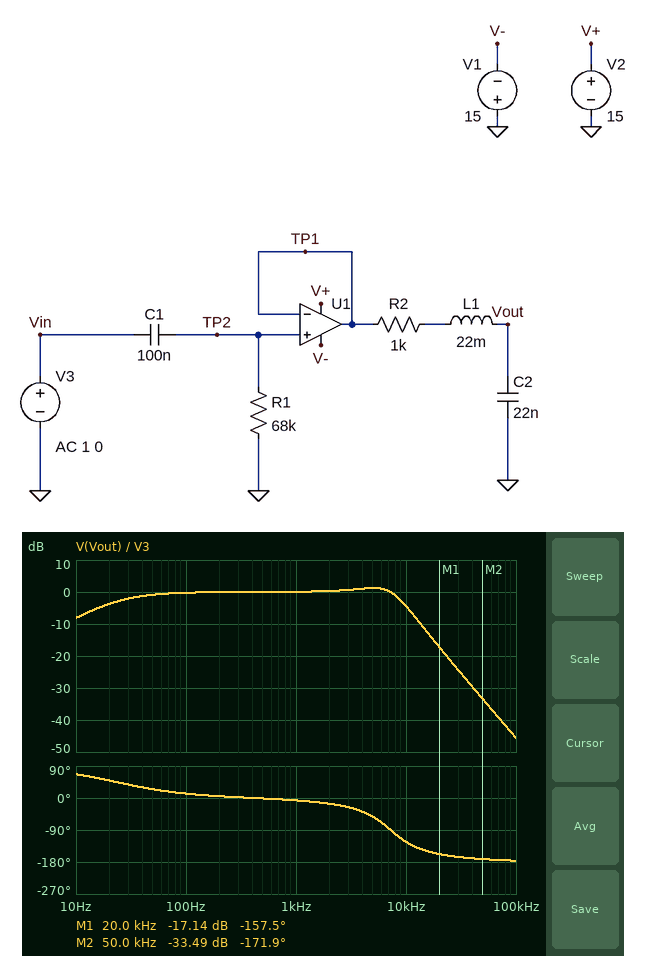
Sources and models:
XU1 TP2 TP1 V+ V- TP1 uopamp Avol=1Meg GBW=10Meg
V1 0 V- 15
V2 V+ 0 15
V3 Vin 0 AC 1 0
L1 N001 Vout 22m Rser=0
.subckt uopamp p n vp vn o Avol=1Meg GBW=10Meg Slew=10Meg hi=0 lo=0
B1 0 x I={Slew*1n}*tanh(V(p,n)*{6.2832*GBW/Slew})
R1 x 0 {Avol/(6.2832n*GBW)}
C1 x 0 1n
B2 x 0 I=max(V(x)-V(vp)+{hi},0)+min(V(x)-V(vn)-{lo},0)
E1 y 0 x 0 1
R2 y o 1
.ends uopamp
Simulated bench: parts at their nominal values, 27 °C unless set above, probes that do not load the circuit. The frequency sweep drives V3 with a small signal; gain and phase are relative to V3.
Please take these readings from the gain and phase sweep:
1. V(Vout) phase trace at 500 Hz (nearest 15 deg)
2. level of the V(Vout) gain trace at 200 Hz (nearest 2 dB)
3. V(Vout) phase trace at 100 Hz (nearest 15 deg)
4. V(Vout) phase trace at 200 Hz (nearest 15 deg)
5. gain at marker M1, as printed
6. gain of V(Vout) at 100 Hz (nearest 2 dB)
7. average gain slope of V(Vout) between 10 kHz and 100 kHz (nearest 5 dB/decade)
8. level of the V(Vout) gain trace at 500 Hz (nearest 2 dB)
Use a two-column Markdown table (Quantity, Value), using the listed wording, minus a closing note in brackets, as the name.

| Quantity | Value |
|---|---|
| V(Vout) phase trace at 500 Hz | 0 deg |
| level of the V(Vout) gain trace at 200 Hz | 0 dB |
| V(Vout) phase trace at 100 Hz | 15 deg |
| V(Vout) phase trace at 200 Hz | 0 deg |
| gain at marker M1, as printed | -17.14 dB |
| gain of V(Vout) at 100 Hz | 0 dB |
| average gain slope of V(Vout) between 10 kHz and 100 kHz | -40 dB/decade |
| level of the V(Vout) gain trace at 500 Hz | 0 dB |
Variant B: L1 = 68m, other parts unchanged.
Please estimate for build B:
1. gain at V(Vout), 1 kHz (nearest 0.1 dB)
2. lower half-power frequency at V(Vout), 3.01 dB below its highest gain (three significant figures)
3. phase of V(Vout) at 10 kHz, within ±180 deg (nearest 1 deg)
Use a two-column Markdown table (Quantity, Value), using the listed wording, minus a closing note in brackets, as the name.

| Quantity | Value |
|---|---|
| gain at V(Vout), 1 kHz | 0.4 dB |
| lower half-power frequency at V(Vout), 3.01 dB below its highest gain | 2.23 kHz |
| phase of V(Vout) at 10 kHz, within ±180 deg | -164 deg |
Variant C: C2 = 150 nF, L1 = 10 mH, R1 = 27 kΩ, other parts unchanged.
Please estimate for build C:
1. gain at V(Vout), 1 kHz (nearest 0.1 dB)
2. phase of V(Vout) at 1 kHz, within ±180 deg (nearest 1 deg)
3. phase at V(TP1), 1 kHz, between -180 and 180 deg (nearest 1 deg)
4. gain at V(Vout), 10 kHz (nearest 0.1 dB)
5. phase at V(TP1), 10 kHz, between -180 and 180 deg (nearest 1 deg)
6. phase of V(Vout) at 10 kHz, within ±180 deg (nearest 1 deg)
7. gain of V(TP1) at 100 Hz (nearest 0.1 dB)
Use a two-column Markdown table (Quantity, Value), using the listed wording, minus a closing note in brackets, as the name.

| Quantity | Value |
|---|---|
| gain at V(Vout), 1 kHz | -2.5 dB |
| phase of V(Vout) at 1 kHz, within ±180 deg | -42 deg |
| phase at V(TP1), 1 kHz, between -180 and 180 deg | 3 deg |
| gain at V(Vout), 10 kHz | -20.5 dB |
| phase at V(TP1), 10 kHz, between -180 and 180 deg | 0 deg |
| phase of V(Vout) at 10 kHz, within ±180 deg | -117 deg |
| gain of V(TP1) at 100 Hz | -1.3 dB |
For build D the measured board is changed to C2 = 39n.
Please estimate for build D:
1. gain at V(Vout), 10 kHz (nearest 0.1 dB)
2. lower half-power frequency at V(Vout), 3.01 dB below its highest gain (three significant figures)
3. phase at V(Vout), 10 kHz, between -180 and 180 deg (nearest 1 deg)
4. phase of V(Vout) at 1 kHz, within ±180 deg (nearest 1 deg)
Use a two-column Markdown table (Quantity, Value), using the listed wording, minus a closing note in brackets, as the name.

| Quantity | Value |
|---|---|
| gain at V(Vout), 10 kHz | -10.7 dB |
| lower half-power frequency at V(Vout), 3.01 dB below its highest gain | 23.7 Hz |
| phase at V(Vout), 10 kHz, between -180 and 180 deg | -134 deg |
| phase of V(Vout) at 1 kHz, within ±180 deg | -13 deg |
